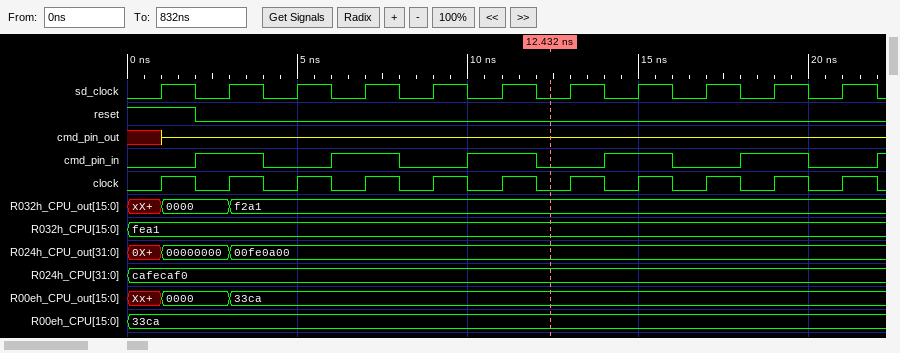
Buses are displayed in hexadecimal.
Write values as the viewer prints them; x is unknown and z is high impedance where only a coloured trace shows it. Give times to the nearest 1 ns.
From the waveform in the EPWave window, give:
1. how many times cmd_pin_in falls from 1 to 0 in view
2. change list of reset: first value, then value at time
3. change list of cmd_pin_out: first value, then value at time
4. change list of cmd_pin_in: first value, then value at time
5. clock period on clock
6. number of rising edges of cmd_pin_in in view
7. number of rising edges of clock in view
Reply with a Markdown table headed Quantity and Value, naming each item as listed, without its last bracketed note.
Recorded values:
| Quantity | Value |
|---|---|
| how many times cmd_pin_in falls from 1 to 0 in view | 5 |
| change list of reset: first value, then value at time | 1, 0 at 2 ns |
| change list of cmd_pin_out: first value, then value at time | x, z at 1 ns |
| change list of cmd_pin_in: first value, then value at time | 0, 1 at 2 ns, 0 at 4 ns, 1 at 6 ns, 0 at 8 ns, 1 at 10 ns, 0 at 12 ns, 1 at 14 ns, 0 at 16 ns, 1 at 18 ns, 0 at 20 ns, 1 at 22 ns |
| clock period on clock | 2 ns |
| number of rising edges of cmd_pin_in in view | 6 |
| number of rising edges of clock in view | 11 |
